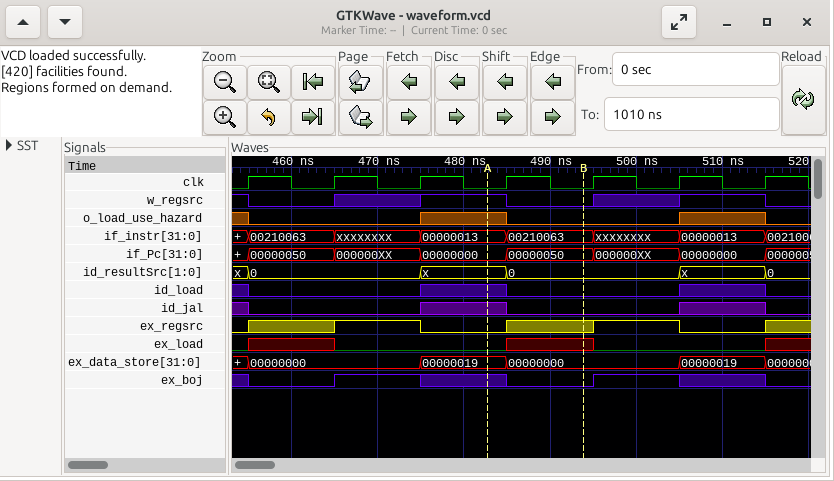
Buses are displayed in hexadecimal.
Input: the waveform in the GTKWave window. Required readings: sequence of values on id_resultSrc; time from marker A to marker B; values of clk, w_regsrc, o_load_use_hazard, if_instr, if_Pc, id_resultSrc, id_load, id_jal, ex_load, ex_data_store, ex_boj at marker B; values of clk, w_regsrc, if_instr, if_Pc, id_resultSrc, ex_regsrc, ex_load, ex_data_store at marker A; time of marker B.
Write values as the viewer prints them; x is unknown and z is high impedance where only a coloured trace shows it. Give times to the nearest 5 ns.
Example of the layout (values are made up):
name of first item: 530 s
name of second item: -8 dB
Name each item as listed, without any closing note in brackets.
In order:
sequence of values on id_resultSrc: x, 0, x, 0, x, 0
time from marker A to marker B: 10 ns
values of clk, w_regsrc, o_load_use_hazard, if_instr, if_Pc, id_resultSrc, id_load, id_jal, ex_load, ex_data_store, ex_boj at marker B: clk=0, w_regsrc=0, o_load_use_hazard=0, if_instr=00210063, if_Pc=00000050, id_resultSrc=0, id_load=0, id_jal=0, ex_load=x, ex_data_store=00000000, ex_boj=0
values of clk, w_regsrc, if_instr, if_Pc, id_resultSrc, ex_regsrc, ex_load, ex_data_store at marker A: clk=0, w_regsrc=1, if_instr=00000013, if_Pc=00000000, id_resultSrc=x, ex_regsrc=0, ex_load=0, ex_data_store=00000019
time of marker B: 495 ns
